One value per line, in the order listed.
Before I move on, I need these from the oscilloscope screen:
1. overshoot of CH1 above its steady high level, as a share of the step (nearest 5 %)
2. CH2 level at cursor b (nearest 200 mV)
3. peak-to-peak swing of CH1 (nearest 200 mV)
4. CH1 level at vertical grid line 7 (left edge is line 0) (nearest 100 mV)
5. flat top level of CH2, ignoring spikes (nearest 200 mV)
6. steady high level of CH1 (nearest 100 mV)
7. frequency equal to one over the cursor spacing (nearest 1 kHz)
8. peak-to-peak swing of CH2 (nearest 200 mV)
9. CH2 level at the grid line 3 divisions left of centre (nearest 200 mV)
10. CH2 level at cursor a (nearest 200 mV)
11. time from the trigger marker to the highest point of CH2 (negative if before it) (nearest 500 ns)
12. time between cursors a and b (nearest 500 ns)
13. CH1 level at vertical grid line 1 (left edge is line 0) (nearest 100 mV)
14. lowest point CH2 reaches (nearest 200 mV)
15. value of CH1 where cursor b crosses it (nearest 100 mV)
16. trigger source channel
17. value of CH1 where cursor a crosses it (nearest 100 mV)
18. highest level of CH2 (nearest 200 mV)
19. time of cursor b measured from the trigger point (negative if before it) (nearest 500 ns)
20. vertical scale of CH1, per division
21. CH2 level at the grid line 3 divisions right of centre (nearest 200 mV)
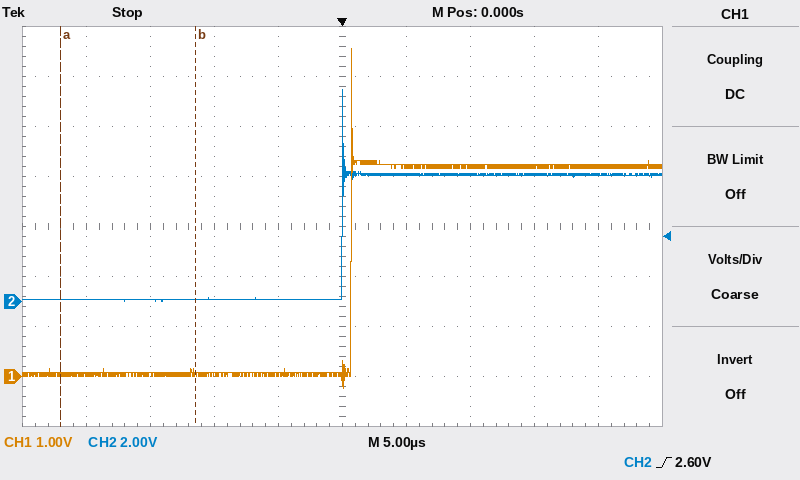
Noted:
55 %
0.0 V
6.8 V
4.2 V
5.0 V
4.2 V
95 kHz
8.4 V
0.0 V
0.0 V
0.0 µs
10.5 µs
0.0 V
0.0 V
100 mV
CH2
0.0 V
8.4 V
-11.5 µs
1 V
5.0 V
